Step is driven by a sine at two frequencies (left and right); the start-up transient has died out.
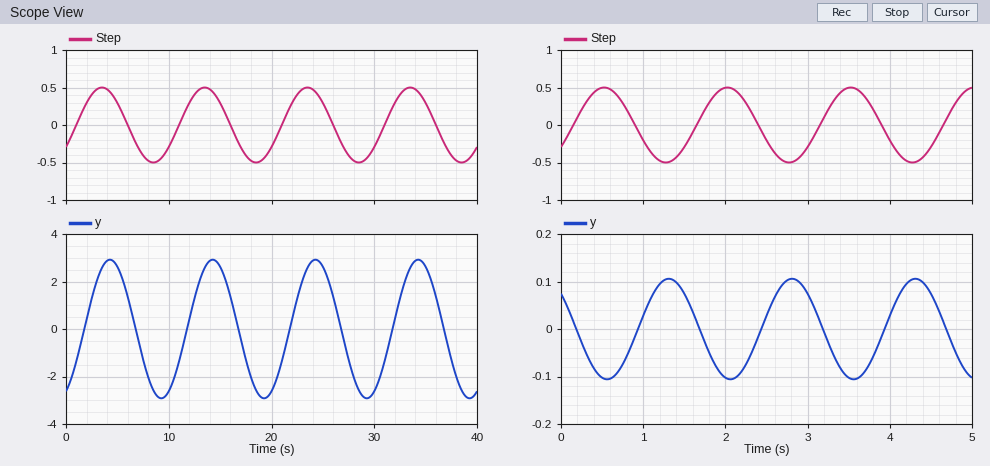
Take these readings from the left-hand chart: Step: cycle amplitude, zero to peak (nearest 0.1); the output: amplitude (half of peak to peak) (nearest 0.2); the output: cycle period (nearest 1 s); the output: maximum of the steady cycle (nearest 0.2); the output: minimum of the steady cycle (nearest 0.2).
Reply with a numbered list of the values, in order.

1. 0.5
2. 3.0
3. 10 s
4. 3.0
5. -3.0
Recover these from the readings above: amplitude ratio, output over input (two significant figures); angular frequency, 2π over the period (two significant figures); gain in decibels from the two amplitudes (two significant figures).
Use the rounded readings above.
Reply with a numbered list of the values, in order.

1. 6.0
2. 0.63 rad/s
3. 16 dB
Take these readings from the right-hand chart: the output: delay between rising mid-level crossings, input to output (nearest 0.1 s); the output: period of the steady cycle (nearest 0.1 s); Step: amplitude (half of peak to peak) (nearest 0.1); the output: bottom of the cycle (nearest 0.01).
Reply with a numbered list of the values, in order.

1. 0.8 s
2. 1.5 s
3. 0.5
4. -0.11
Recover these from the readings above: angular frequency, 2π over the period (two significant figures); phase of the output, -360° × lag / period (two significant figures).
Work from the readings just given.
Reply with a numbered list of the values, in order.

1. 4.2 rad/s
2. -190°
